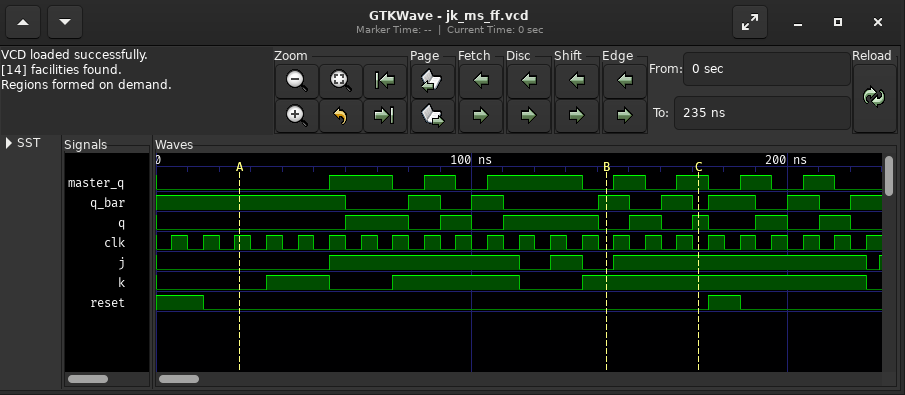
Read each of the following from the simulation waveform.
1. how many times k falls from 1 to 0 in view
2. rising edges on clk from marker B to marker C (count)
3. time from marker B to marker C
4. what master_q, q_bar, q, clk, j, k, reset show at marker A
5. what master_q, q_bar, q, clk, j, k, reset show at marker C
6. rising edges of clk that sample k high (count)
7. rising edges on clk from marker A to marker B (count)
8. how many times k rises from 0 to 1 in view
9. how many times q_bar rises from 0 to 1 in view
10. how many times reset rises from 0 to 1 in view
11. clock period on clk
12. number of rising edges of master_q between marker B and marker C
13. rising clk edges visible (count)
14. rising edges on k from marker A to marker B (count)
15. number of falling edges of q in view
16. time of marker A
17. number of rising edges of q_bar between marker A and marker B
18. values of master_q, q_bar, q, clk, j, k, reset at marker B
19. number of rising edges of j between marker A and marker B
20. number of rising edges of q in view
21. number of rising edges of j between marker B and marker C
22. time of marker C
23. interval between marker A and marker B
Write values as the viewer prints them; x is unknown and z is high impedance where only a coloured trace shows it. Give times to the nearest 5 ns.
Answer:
3
3
30 ns
master_q=0, q_bar=1, q=0, clk=1, j=0, k=0, reset=0
master_q=1, q_bar=0, q=1, clk=0, j=1, k=1, reset=0
15
11
3
7
1
10 ns
2
23
3
7
25 ns
3
master_q=0, q_bar=1, q=0, clk=0, j=0, k=1, reset=0
2
7
1
170 ns
115 ns
